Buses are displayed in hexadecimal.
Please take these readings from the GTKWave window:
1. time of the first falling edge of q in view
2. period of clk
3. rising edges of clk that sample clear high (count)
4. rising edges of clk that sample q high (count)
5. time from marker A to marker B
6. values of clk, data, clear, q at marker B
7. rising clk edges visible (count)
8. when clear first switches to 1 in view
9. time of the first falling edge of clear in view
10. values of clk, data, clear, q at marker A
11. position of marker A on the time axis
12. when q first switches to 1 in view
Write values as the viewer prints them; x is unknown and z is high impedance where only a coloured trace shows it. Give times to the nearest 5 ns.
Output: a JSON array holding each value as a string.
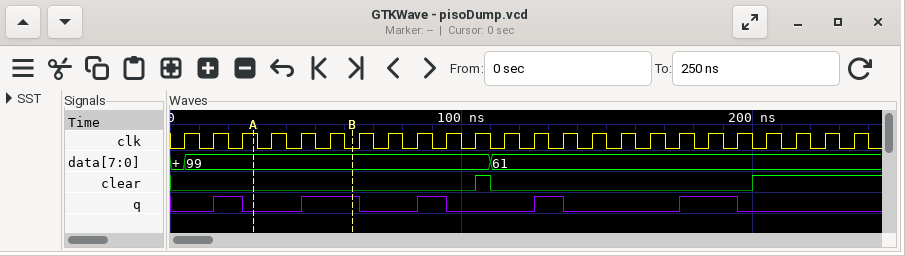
["25 ns", "10 ns", "4", "7", "35 ns", "clk=0, data=99, clear=0, q=1", "24", "105 ns", "110 ns", "clk=1, data=99, clear=0, q=0", "30 ns", "15 ns"]
